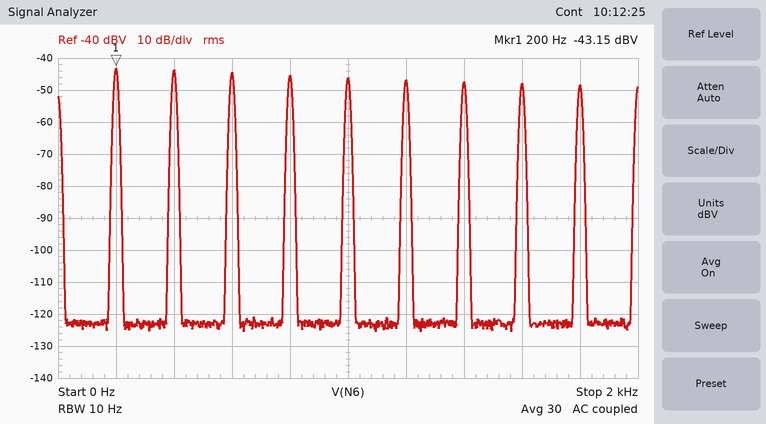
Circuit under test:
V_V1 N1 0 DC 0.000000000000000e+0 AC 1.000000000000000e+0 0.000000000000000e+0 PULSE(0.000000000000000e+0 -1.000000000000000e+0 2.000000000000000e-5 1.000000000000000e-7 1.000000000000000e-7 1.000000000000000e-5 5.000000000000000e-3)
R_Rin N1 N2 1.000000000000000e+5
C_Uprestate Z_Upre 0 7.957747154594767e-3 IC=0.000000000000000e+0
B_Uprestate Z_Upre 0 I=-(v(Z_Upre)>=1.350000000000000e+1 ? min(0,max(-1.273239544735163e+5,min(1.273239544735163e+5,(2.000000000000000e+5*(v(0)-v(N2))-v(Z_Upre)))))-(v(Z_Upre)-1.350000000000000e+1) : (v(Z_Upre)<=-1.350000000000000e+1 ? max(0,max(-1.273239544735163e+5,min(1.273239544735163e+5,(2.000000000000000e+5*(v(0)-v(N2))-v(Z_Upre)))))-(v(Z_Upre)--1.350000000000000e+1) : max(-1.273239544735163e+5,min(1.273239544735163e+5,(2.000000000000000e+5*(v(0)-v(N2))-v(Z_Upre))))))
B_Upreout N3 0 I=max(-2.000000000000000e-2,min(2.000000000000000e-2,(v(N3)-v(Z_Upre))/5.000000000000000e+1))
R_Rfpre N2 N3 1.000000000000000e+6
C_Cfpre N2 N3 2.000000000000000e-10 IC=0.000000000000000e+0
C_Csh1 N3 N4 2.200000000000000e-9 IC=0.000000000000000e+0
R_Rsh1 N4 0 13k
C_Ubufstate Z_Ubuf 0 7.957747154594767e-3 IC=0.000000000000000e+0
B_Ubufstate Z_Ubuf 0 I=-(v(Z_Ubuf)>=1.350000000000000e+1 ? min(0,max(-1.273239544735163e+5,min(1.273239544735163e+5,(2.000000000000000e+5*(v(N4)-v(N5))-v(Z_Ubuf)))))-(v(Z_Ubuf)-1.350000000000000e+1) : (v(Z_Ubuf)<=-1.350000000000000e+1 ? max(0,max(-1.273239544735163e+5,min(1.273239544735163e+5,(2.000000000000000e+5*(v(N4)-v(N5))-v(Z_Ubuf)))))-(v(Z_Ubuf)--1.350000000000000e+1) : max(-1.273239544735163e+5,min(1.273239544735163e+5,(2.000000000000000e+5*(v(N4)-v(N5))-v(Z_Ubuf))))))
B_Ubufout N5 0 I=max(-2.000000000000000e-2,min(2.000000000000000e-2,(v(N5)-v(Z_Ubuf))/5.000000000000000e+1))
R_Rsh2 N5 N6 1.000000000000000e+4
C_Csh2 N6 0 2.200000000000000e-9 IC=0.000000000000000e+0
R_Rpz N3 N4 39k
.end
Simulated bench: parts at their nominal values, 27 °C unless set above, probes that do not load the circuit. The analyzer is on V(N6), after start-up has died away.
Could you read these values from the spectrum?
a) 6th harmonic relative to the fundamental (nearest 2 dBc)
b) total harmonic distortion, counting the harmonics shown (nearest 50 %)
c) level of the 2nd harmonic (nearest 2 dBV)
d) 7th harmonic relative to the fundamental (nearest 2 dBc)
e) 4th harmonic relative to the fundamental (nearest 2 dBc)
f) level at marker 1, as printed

-4 dBc
200 %
-44 dBV
-4 dBc
-2 dBc
-43.15 dBV
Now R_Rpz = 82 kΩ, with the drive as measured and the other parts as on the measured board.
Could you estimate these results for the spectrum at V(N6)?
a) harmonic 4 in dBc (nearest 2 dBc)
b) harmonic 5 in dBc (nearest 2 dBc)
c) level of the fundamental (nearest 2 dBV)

0 dBc
0 dBc
-48 dBV
